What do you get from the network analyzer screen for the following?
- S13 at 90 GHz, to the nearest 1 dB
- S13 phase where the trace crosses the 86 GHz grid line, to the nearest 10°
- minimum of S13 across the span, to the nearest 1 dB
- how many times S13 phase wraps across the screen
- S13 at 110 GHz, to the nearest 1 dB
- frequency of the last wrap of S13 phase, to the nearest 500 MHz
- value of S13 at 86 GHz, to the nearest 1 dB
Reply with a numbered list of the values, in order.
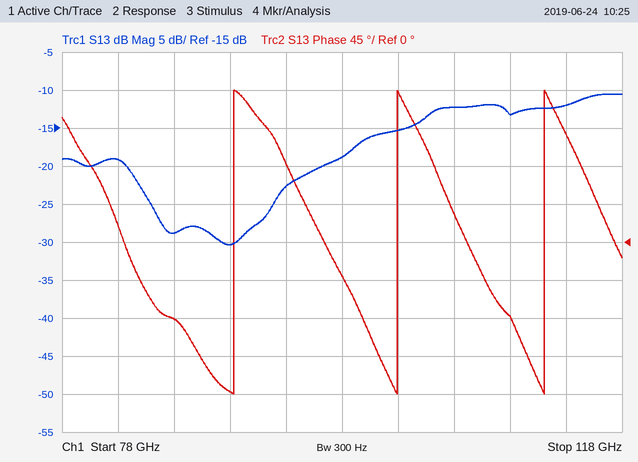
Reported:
1. -30 dB
2. -90°
3. -30 dB
4. 3
5. -13 dB
6. 112.5 GHz
7. -29 dB
